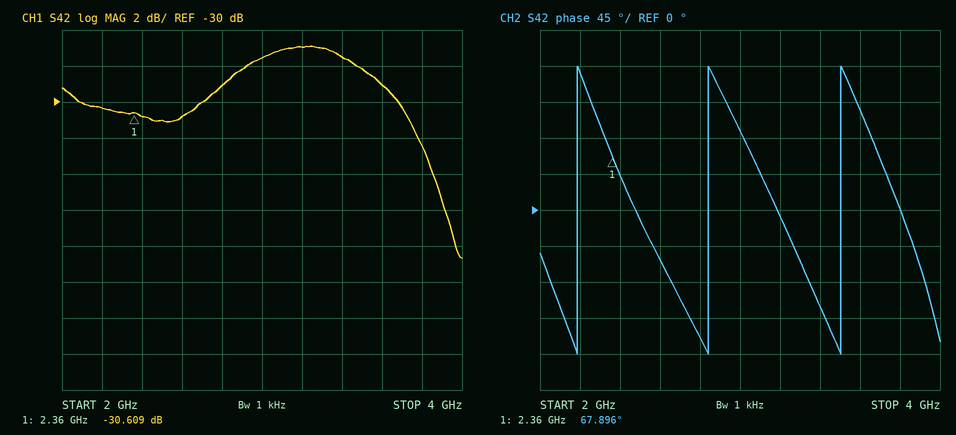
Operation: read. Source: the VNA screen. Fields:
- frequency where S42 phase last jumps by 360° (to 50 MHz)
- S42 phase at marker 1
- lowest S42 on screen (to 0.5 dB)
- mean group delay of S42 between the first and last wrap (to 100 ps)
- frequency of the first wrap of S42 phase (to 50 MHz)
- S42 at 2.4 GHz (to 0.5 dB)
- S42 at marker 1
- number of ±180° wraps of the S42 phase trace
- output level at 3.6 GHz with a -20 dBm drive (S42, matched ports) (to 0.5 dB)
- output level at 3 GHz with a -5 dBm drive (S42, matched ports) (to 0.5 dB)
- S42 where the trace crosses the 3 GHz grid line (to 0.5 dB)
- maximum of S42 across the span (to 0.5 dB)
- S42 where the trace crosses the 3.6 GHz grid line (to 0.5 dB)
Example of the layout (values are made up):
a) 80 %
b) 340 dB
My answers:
a) 3.50 GHz
b) 67.896°
c) -38.5 dB
d) 1.5 ns
e) 2.20 GHz
f) -31.0 dB
g) -30.609 dB
h) 3
i) -49.0 dBm
j) -32.5 dBm
k) -27.5 dB
l) -27.0 dB
m) -29.0 dB
